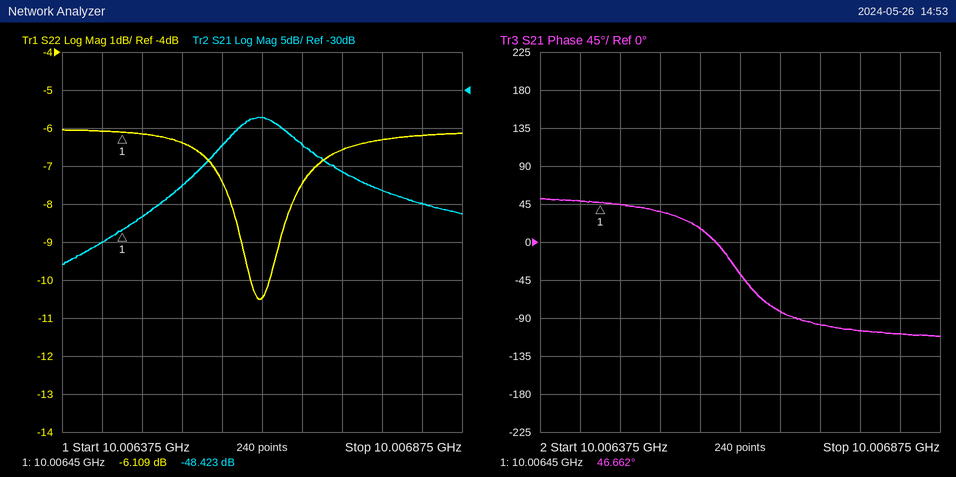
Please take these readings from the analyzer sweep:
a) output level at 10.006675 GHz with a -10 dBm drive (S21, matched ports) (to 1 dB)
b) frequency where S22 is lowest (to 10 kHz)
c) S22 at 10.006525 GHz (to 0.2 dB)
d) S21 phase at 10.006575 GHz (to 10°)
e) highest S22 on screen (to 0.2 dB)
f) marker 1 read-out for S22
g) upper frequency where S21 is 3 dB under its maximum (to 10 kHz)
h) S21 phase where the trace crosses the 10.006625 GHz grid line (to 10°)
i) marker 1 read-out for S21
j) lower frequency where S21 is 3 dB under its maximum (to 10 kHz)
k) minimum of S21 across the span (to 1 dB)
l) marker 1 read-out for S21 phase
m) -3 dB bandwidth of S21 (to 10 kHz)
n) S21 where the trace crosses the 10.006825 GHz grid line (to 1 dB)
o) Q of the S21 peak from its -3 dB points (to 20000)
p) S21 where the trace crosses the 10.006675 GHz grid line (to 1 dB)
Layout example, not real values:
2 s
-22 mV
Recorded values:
-47 dBm
10.00662 GHz
-6.4 dB
20°
-6.0 dB
-6.109 dB
10.00667 GHz
-40°
-48.423 dB
10.00658 GHz
-53 dB
46.662°
90 kHz
-45 dB
120000
-37 dB
